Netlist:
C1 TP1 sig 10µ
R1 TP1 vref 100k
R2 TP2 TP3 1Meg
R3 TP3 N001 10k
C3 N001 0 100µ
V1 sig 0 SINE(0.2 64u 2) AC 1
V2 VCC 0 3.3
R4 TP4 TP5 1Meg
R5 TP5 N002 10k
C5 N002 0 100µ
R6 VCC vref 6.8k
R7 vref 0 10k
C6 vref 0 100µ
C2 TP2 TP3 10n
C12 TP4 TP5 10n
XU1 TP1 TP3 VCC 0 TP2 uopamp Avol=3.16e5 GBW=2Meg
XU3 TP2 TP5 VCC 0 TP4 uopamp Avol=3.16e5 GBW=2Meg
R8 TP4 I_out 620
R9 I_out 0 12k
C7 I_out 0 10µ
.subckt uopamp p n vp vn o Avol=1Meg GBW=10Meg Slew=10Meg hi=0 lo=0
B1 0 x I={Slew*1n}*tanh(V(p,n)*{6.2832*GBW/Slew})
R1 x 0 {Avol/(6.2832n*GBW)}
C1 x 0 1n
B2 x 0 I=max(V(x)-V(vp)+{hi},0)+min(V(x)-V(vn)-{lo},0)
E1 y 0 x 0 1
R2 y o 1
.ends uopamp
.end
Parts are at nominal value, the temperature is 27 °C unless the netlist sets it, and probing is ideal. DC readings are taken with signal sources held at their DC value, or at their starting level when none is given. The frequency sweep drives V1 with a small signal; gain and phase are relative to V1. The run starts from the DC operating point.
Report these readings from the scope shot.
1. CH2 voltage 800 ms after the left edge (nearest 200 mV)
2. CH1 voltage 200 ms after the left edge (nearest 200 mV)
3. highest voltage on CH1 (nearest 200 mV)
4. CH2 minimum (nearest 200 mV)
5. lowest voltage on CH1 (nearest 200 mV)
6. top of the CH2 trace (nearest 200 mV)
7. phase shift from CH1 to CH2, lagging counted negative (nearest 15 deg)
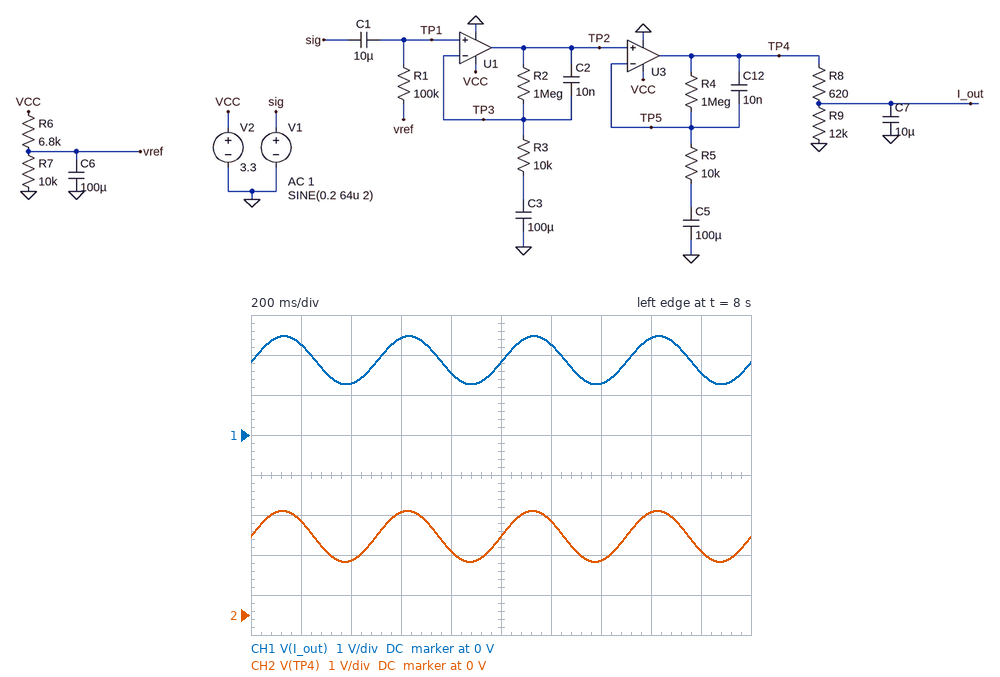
1.6 V
2.2 V
2.4 V
1.4 V
1.2 V
2.6 V
0 deg
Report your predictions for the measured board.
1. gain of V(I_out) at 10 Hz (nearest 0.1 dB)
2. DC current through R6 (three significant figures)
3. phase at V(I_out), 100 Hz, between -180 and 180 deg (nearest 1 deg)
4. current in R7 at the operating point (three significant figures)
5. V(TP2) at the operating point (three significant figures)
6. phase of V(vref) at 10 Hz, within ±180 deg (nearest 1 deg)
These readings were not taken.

76.3 dB
196 µA
131 deg
196 µA
1.96 V
-87 deg
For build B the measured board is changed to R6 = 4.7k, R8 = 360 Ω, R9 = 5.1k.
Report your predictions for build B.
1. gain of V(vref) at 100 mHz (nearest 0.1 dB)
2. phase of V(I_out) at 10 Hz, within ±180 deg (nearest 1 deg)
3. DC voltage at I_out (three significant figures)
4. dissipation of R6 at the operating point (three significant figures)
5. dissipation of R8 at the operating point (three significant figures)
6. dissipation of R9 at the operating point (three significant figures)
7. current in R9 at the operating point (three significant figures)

-35.7 dB
-73 deg
2.10 V
237 µW
60.9 µW
862 µW
411 µA
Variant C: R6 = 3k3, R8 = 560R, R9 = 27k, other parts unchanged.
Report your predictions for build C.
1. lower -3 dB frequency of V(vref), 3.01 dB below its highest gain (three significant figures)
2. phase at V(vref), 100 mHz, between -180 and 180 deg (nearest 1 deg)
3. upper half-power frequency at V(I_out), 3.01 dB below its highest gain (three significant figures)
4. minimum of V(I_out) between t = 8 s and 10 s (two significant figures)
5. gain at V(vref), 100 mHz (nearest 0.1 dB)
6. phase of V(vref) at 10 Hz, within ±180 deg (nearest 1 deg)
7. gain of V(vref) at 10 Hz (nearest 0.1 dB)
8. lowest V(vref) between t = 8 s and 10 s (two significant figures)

110 mHz
48 deg
9.76 Hz
1.8 V
-37.8 dB
-85 deg
-56.0 dB
2.5 V
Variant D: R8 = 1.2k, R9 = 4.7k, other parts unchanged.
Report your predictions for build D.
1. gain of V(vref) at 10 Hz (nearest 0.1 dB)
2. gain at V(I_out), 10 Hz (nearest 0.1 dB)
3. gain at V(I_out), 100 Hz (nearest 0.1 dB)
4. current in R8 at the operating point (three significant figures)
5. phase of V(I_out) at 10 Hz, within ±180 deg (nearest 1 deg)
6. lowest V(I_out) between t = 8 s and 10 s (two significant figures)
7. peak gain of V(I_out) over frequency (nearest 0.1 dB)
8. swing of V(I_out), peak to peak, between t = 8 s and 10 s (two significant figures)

-56.0 dB
74.0 dB
30.4 dB
333 µA
-92 deg
1.1 V
77.9 dB
1.0 V
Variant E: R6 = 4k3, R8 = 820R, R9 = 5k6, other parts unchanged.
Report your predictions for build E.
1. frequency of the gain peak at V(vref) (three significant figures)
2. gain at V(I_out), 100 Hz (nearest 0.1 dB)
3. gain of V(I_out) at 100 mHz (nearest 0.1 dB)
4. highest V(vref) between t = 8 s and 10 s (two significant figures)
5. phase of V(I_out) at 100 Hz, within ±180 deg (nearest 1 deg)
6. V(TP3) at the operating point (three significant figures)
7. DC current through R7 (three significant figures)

290 mHz
33.6 dB
62.7 dB
2.3 V
128 deg
2.31 V
231 µA
